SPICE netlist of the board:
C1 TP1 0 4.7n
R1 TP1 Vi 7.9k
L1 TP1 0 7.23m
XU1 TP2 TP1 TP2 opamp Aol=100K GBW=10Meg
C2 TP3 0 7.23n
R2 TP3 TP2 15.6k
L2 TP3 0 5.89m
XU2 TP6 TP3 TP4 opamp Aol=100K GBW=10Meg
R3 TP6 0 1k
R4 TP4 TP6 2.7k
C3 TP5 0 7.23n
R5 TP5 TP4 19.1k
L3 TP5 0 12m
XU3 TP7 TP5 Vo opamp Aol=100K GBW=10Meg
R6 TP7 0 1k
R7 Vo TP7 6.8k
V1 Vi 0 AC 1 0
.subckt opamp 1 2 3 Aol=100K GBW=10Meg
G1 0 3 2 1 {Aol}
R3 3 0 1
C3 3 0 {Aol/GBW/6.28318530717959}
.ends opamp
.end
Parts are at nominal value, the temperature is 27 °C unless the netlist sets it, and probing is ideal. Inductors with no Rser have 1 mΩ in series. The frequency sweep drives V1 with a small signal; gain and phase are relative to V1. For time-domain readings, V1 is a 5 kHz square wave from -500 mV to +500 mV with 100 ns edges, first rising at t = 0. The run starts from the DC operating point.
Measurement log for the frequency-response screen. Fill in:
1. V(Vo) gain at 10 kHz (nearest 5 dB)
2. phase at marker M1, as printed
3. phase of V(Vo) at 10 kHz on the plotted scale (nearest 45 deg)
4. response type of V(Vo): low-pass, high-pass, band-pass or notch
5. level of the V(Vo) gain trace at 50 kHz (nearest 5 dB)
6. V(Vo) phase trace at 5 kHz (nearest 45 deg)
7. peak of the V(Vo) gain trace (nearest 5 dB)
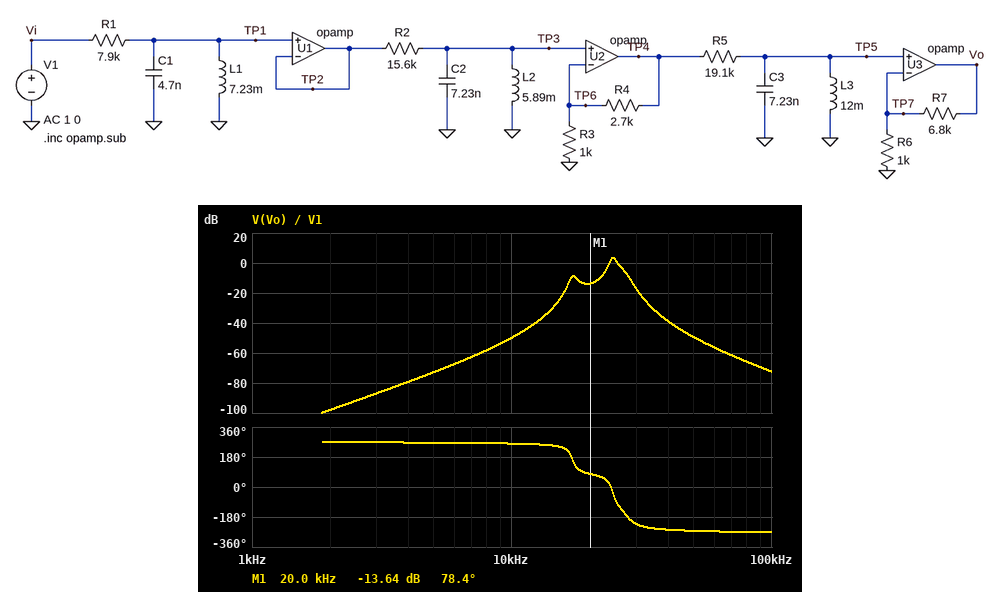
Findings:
-50 dB
78.4 deg
270 deg
band-pass
-50 dB
270 deg
5 dB
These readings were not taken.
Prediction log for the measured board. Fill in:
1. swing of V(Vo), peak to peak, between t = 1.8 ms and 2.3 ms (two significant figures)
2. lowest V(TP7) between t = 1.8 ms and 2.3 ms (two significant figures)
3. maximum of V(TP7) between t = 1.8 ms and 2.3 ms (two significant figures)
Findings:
330 mV
-21 mV
21 mV
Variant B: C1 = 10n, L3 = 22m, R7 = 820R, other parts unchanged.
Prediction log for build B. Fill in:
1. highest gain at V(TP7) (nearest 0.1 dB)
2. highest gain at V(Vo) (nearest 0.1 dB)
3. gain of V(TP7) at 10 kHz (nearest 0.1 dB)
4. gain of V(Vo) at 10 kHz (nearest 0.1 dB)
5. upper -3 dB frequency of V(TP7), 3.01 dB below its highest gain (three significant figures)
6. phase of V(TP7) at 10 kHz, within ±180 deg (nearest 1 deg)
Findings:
-26.5 dB
-21.3 dB
-55.8 dB
-50.6 dB
24.9 kHz
-108 deg
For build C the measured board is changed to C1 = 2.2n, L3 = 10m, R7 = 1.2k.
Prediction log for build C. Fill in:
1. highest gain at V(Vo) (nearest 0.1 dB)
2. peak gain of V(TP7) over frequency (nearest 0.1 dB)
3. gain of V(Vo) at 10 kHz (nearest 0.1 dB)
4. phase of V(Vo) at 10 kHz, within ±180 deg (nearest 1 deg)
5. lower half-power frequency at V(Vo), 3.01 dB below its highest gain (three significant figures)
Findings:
-13.8 dB
-20.7 dB
-63.7 dB
-98 deg
23.6 kHz
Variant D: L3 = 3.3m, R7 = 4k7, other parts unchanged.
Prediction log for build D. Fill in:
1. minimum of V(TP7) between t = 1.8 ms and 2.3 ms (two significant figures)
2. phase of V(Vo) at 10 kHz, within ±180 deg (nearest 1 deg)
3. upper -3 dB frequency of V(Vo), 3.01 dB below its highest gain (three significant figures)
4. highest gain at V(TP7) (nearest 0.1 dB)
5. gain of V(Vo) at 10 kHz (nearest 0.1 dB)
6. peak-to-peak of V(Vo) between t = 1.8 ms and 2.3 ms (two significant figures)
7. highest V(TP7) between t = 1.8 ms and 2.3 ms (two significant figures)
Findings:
-17 mV
-97 deg
33.0 kHz
-16.6 dB
-66.4 dB
200 mV
17 mV
